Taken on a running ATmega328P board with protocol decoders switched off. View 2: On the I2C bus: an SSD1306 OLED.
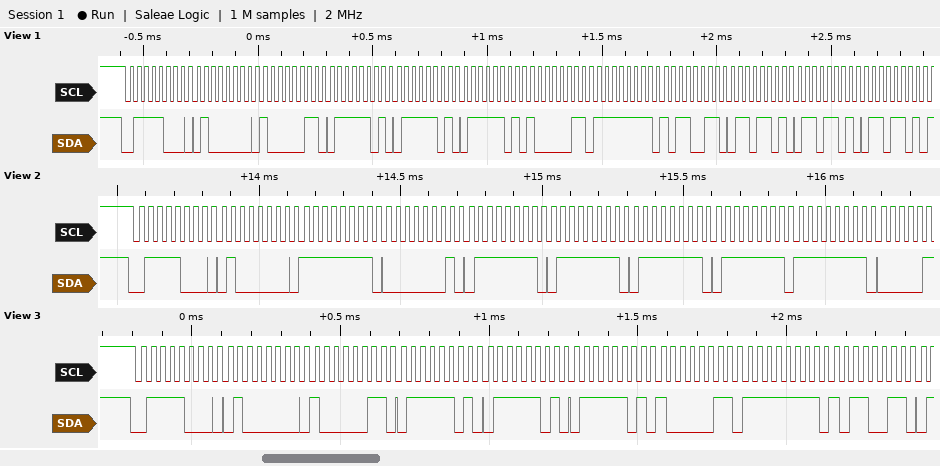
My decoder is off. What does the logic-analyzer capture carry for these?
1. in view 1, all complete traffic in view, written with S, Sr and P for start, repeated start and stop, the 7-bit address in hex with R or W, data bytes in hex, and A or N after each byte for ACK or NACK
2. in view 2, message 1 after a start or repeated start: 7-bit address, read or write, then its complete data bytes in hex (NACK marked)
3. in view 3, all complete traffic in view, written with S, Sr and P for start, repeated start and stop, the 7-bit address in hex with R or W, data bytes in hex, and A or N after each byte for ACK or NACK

S 3CW A 40 A 83 A 7D A 7D A 7D A 83 A FF A B3 A 6D A 6D A 6D A
0x3C write: 40 FF 01 7F 7F 7F 7F FF
S 3CW A 40 A 83 A 7D A 7D A 7D A 83 A FF A B3 A
